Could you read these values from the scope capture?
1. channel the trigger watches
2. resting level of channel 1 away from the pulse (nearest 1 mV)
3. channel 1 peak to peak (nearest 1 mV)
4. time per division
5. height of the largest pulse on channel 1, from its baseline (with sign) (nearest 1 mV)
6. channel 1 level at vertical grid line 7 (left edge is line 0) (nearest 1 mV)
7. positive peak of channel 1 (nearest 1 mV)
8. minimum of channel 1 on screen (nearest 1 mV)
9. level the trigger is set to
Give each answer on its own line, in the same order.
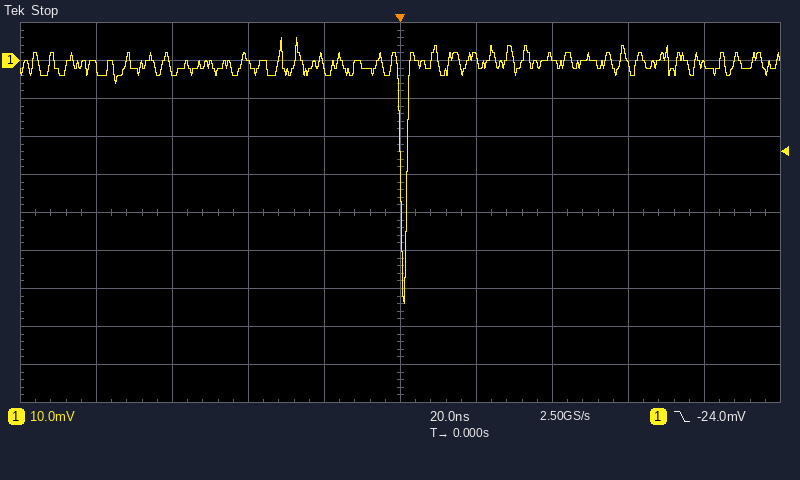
channel 1
-1 mV
70 mV
20 ns
-63 mV
1 mV
6 mV
-64 mV
-24.0 mV
